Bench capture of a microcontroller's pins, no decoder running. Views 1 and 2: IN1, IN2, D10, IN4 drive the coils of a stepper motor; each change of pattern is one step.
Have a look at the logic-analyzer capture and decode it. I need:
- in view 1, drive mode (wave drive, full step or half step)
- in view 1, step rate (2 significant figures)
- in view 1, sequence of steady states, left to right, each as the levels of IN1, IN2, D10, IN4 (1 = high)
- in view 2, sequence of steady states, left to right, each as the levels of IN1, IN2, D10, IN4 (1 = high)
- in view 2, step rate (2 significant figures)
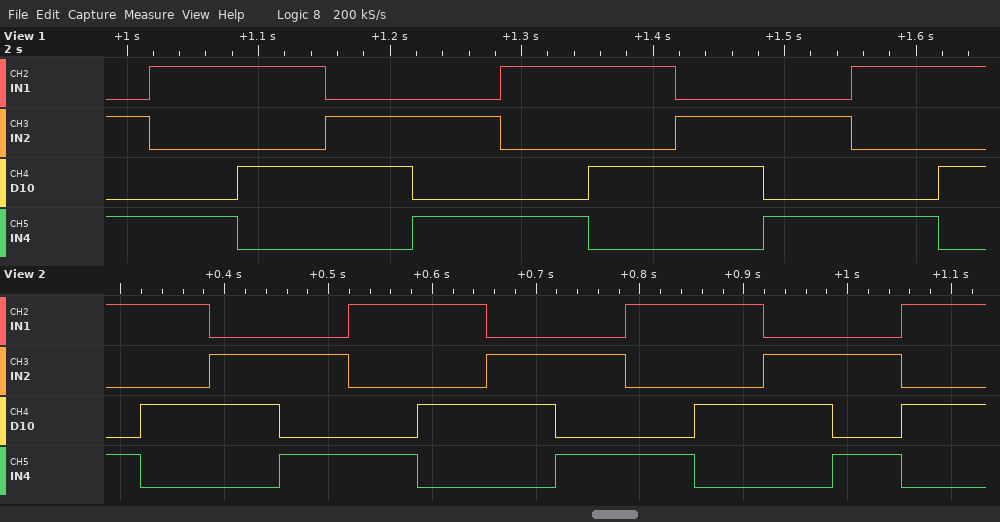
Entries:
full step
15 steps/s
0101 1001 1010 0110 0101 1001 1010 0110 0101 1001 1010
1001 1010 0110 0101 1001 1010 0110 0101 1001 1010 0110 0101 1010
15 steps/s
